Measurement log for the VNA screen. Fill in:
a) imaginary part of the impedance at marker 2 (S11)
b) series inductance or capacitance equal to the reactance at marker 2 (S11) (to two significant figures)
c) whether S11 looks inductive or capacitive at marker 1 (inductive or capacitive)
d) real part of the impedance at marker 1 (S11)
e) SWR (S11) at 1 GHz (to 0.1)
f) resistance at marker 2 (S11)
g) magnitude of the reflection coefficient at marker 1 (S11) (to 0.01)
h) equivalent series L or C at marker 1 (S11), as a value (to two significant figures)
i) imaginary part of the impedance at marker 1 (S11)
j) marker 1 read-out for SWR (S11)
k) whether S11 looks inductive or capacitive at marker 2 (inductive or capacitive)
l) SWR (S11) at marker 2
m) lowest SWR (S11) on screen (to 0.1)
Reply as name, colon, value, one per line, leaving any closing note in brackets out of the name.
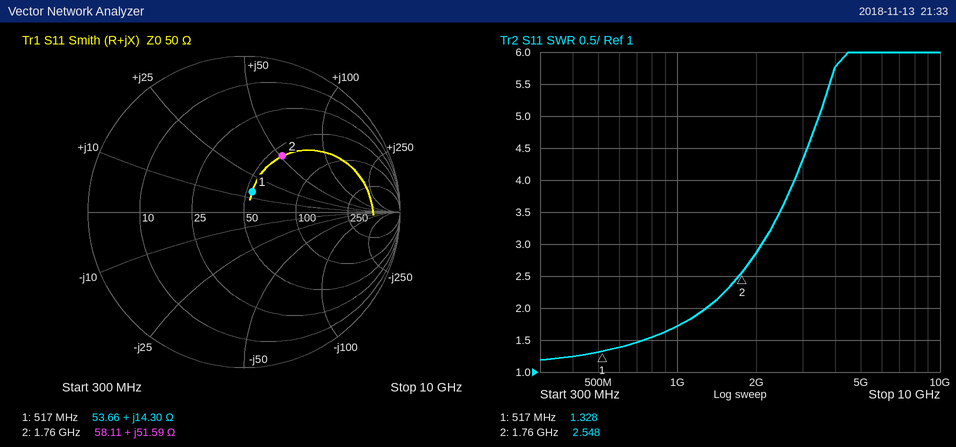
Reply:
imaginary part of the impedance at marker 2: +51.59 Ω
series inductance or capacitance equal to the reactance at marker 2 (S11): 4.7 nH
whether S11 looks inductive or capacitive at marker 1: inductive
real part of the impedance at marker 1: 53.66 Ω
SWR (S11) at 1 GHz: 1.7
resistance at marker 2: 58.11 Ω
magnitude of the reflection coefficient at marker 1 (S11): 0.14
equivalent series L or C at marker 1 (S11), as a value: 4.4 nH
imaginary part of the impedance at marker 1: +14.30 Ω
marker 1 read-out for SWR: 1.328
whether S11 looks inductive or capacitive at marker 2: inductive
SWR (S11) at marker 2: 2.548
lowest SWR (S11) on screen: 1.2
